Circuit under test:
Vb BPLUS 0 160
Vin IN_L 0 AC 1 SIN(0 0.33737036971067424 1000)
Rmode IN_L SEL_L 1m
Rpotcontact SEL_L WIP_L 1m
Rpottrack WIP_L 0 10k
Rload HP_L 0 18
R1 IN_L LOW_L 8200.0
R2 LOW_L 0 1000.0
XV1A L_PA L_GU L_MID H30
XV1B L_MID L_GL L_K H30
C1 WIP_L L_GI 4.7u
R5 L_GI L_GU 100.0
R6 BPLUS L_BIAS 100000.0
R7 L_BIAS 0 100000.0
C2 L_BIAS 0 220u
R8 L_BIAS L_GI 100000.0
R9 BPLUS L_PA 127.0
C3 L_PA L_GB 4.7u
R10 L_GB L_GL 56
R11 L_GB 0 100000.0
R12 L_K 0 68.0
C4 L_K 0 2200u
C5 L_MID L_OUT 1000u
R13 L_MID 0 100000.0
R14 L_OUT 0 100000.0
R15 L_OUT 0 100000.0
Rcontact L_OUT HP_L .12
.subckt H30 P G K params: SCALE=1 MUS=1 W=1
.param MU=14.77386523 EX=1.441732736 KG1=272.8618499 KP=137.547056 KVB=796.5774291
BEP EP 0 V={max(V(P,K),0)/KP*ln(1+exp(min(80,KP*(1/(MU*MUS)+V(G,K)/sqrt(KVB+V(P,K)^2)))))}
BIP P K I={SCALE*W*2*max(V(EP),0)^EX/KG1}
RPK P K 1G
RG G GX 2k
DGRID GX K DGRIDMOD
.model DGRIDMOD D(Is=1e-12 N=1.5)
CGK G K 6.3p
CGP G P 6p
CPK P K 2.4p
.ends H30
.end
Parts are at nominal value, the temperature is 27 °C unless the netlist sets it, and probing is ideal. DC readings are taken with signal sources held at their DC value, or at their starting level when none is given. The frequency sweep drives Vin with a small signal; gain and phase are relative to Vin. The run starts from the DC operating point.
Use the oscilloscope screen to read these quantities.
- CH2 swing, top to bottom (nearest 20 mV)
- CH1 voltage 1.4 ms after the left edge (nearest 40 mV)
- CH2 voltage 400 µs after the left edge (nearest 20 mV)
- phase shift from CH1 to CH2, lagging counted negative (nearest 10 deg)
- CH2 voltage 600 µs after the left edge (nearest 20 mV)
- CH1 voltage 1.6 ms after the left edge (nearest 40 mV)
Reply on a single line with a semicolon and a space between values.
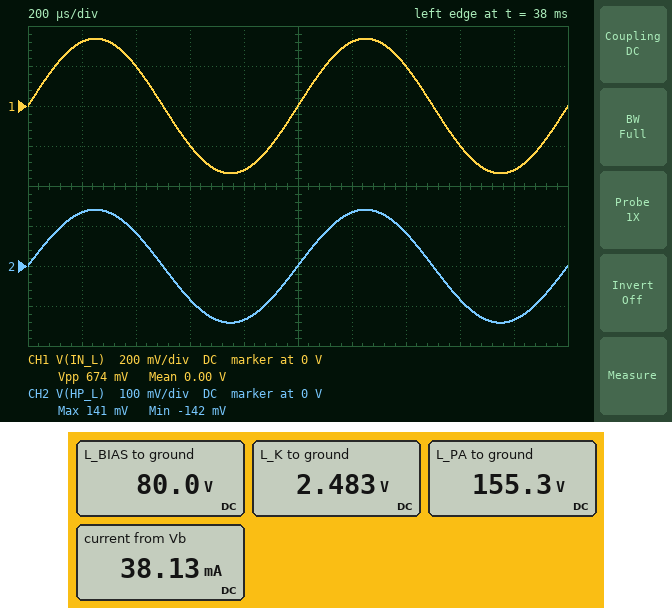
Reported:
280 mV; 200 mV; 80 mV; 0 deg; -80 mV; -200 mV
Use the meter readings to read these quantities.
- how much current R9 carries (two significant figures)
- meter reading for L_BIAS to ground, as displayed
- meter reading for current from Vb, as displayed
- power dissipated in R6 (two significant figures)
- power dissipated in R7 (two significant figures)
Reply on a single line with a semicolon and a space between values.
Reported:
37 mA; 80.0 V; 38.13 mA; 64 mW; 64 mW
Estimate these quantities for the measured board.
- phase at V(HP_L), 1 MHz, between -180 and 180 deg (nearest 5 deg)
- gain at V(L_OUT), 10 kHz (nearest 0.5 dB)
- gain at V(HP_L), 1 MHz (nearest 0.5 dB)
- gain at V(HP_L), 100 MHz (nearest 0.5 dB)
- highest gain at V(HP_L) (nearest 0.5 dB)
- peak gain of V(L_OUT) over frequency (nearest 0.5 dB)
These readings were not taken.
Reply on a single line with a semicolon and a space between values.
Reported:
0 deg; -7.5 dB; -7.5 dB; -17.0 dB; -7.5 dB; -7.5 dB
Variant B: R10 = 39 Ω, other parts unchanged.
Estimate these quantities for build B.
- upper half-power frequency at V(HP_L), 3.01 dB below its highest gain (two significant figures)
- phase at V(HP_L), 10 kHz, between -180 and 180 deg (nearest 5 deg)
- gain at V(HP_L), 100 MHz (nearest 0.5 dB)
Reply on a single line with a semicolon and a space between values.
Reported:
51 MHz; 0 deg; -16.5 dB
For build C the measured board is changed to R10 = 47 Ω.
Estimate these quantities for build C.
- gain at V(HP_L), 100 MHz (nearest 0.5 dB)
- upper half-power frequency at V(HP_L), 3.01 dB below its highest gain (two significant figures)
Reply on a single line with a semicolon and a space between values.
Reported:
-16.5 dB; 50 MHz
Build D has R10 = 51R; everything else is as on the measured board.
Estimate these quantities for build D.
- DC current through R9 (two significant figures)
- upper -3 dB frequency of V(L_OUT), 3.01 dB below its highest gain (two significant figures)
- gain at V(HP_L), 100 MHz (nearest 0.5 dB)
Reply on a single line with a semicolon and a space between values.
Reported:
37 mA; 50 MHz; -16.5 dB
